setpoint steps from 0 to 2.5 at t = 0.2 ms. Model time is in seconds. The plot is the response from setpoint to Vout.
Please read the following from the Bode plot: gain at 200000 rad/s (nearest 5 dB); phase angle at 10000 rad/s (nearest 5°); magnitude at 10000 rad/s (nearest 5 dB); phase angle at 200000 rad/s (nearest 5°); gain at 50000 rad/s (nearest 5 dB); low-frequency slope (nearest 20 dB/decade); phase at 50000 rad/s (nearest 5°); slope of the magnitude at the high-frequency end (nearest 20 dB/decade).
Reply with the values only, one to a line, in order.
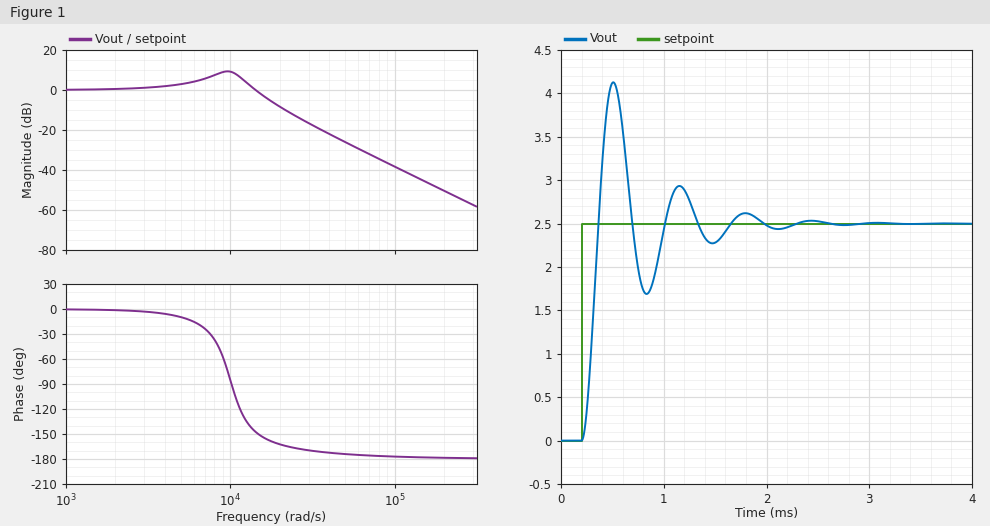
-50 dB
-85°
10 dB
-180°
-25 dB
0 dB/decade
-175°
-40 dB/decade
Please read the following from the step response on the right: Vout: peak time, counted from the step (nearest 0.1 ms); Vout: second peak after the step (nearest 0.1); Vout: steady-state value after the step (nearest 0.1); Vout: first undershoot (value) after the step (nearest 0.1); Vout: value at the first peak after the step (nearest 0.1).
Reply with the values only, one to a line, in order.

0.3 ms
2.9
2.5
1.7
4.1
